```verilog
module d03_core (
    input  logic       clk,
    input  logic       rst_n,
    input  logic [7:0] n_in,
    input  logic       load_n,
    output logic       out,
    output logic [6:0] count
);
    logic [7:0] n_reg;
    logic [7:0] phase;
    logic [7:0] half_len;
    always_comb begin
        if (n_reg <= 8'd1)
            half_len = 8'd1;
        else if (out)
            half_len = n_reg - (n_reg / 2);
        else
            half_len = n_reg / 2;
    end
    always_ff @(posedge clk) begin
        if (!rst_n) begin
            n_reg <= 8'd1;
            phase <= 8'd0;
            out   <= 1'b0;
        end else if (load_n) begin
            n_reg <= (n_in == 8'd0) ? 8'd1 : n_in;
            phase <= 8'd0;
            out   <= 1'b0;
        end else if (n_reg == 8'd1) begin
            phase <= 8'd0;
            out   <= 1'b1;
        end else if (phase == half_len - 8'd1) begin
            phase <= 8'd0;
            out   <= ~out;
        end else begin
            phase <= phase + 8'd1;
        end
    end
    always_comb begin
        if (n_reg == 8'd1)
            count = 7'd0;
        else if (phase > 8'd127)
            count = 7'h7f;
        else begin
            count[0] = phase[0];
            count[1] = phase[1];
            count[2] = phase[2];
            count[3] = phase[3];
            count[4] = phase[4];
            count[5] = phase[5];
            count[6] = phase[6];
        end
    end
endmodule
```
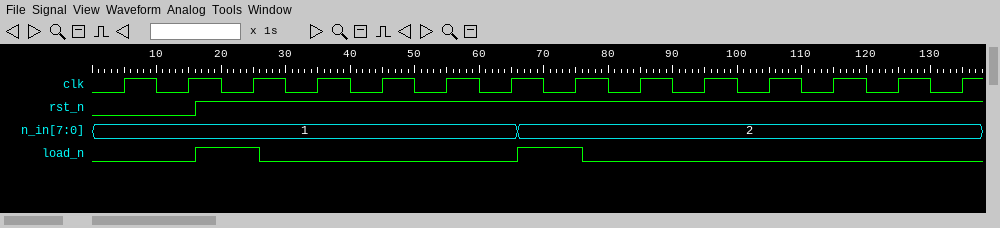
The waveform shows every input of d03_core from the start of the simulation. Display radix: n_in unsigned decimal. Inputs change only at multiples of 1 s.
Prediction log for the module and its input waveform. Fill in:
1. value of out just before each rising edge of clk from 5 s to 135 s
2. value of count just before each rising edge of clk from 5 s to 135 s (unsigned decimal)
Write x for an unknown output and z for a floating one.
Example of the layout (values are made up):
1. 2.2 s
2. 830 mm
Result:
1. x 0 0 0 1 1 1 1 0 1 0 1 0 1
2. x, 0, 0, 0, 0, 0, 0, 0, 0, 0, 0, 0, 0, 0
